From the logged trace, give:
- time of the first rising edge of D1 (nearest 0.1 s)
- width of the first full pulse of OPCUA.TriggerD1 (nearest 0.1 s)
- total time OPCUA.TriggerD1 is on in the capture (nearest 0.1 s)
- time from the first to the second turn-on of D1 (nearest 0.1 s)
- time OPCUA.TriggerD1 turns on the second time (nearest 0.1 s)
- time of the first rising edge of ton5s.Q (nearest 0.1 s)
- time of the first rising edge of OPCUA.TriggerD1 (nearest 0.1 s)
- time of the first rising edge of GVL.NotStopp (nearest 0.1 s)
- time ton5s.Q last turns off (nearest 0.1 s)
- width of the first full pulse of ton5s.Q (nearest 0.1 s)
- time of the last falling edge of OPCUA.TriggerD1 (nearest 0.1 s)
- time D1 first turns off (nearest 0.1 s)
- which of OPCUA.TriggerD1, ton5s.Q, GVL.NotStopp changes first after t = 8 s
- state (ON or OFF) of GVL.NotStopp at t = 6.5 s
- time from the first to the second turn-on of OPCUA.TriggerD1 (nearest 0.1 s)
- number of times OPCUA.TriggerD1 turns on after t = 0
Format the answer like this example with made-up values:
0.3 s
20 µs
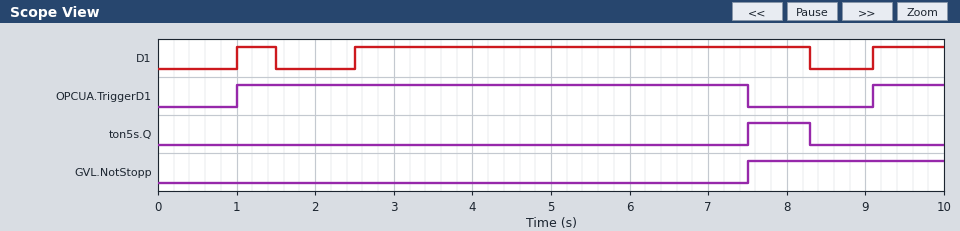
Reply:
1.0 s
6.5 s
7.4 s
1.5 s
9.1 s
7.5 s
1.0 s
7.5 s
8.3 s
0.8 s
7.5 s
1.5 s
ton5s.Q
OFF
8.1 s
2
